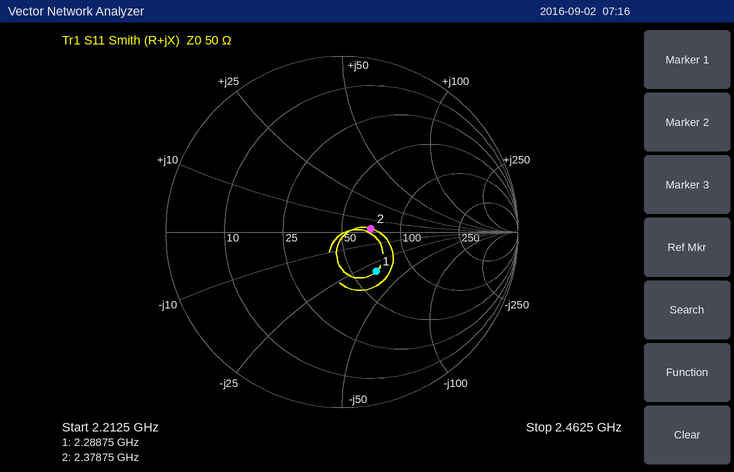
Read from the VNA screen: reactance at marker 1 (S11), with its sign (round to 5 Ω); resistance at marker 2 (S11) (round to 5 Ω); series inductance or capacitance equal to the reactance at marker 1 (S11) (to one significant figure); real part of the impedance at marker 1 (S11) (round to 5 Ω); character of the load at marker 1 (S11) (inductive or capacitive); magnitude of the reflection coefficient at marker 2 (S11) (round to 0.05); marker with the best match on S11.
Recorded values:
-30 Ω
70 Ω
2 pF
65 Ω
capacitive
0.15
marker 2
